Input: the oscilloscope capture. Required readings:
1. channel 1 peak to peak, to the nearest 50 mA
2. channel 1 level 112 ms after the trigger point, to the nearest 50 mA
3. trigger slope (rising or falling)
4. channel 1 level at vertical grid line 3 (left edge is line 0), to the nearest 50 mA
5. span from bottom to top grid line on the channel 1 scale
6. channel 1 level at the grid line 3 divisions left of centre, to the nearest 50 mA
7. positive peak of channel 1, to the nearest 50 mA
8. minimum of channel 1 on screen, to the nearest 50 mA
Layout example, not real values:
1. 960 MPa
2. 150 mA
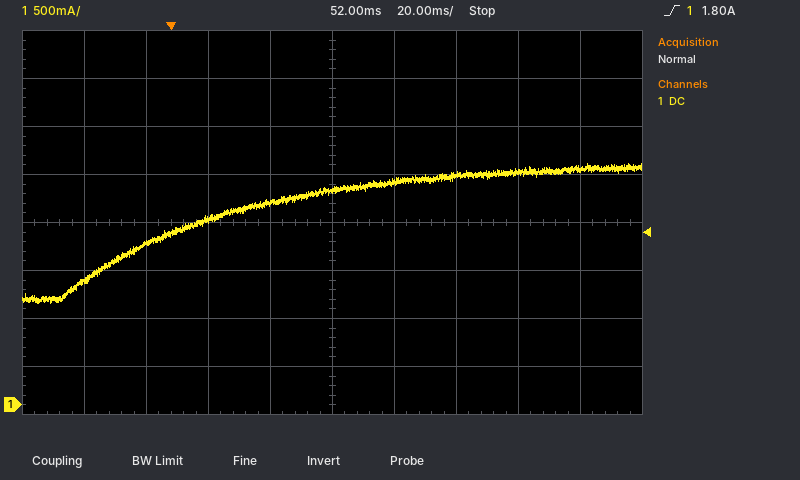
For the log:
1. 1.45 A
2. 2.45 A
3. rising
4. 1.95 A
5. 4 A
6. 1.70 A
7. 2.50 A
8. 1.05 A
